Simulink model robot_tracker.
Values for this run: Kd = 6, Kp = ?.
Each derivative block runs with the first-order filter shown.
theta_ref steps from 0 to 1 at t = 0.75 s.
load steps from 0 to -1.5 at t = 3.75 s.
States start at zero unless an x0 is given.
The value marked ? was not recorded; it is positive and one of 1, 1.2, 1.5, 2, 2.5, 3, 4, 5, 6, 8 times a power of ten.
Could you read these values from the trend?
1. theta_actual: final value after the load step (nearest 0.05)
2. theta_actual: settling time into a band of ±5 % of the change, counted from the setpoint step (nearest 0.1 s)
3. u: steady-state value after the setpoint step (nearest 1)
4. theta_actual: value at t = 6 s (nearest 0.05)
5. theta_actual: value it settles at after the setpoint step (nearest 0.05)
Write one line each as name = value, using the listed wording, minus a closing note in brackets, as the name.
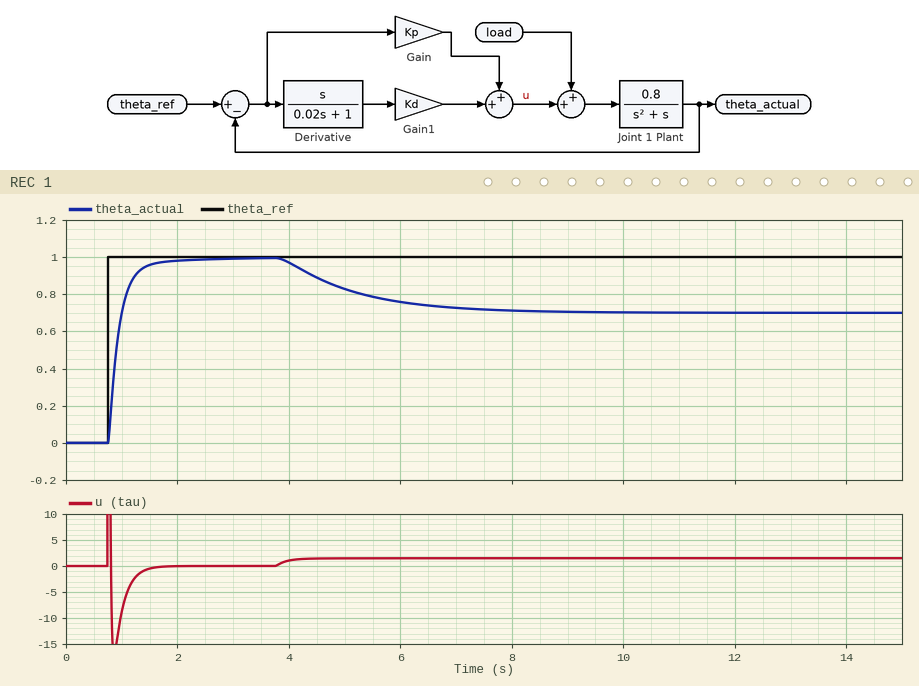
theta_actual: final value after the load step = 0.70
theta_actual: settling time into a band of ±5 % of the change, counted from the setpoint step = 0.7 s
u: steady-state value after the setpoint step = 0
theta_actual: value at t = 6 s = 0.75
theta_actual: value it settles at after the setpoint step = 1.00
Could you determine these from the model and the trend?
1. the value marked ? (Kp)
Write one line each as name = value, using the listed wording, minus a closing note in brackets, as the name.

the value marked ? = 5
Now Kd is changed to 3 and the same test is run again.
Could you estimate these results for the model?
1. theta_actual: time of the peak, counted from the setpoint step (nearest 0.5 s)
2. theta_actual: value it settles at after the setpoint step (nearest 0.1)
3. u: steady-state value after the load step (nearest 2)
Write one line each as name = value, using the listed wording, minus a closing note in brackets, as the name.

theta_actual: time of the peak, counted from the setpoint step = 1.5 s
theta_actual: value it settles at after the setpoint step = 1.0
u: steady-state value after the load step = 2
